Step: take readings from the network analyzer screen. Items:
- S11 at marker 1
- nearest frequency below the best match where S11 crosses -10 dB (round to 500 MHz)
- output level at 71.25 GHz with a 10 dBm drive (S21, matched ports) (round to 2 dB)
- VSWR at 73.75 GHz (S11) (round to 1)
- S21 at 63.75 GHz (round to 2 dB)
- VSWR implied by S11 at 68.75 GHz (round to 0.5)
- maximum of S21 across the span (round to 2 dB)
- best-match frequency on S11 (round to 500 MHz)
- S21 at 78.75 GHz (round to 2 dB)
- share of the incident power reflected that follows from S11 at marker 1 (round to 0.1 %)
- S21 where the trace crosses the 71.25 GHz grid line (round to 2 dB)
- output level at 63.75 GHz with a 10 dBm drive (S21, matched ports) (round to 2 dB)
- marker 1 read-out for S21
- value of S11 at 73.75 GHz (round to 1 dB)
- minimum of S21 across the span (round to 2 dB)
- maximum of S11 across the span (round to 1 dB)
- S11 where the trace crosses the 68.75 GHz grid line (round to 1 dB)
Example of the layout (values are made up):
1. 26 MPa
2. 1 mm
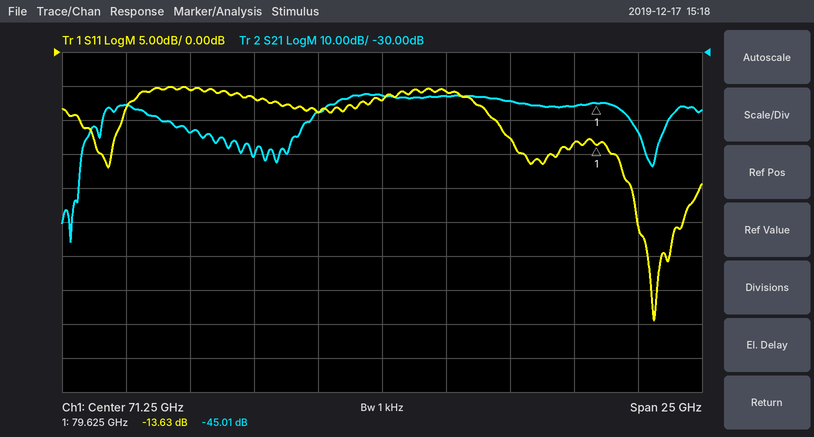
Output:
1. -13.63 dB
2. 75.5 GHz
3. -32 dBm
4. 3
5. -54 dB
6. 2.0
7. -42 dB
8. 82.0 GHz
9. -46 dB
10. 4.3 %
11. -42 dB
12. -44 dBm
13. -45.01 dB
14. -6 dB
15. -86 dB
16. -5 dB
17. -9 dB
